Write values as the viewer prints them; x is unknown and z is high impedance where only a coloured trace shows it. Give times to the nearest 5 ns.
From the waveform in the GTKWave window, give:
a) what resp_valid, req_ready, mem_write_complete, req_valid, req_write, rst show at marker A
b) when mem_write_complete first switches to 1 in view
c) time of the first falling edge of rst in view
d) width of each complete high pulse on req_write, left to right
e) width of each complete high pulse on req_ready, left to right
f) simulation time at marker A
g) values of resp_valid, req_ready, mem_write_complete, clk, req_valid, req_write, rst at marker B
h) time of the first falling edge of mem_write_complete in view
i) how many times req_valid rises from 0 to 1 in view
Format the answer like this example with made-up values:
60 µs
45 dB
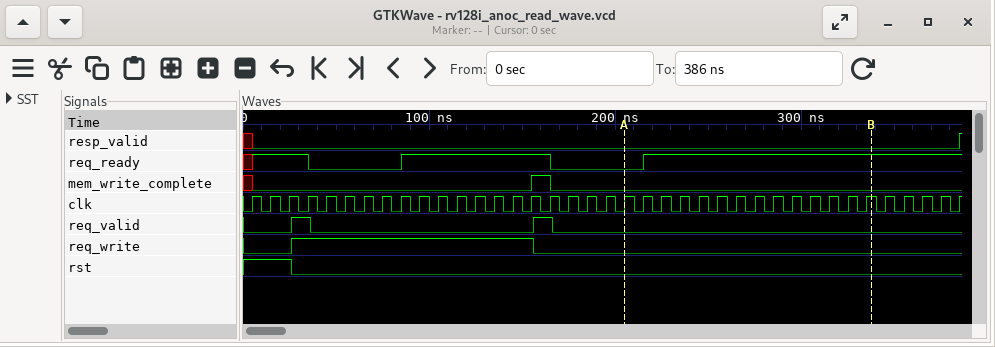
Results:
resp_valid=0, req_ready=0, mem_write_complete=0, req_valid=0, req_write=0, rst=0
155 ns
25 ns
130 ns
80 ns
205 ns
resp_valid=0, req_ready=1, mem_write_complete=0, clk=1, req_valid=0, req_write=0, rst=0
165 ns
2
